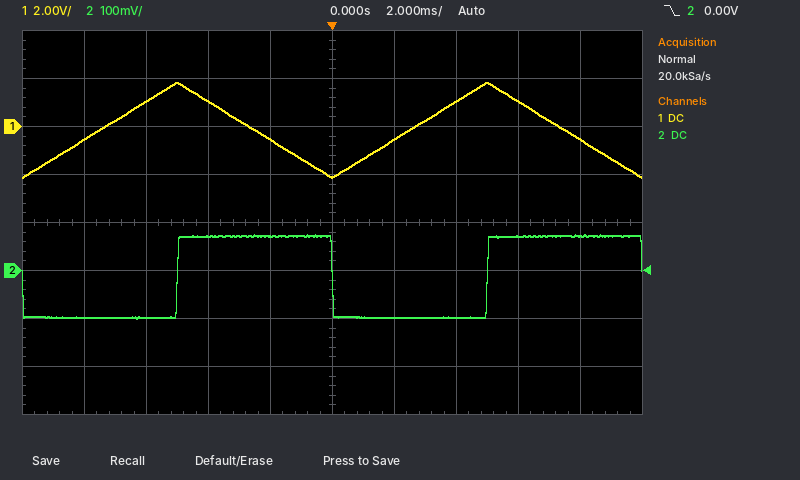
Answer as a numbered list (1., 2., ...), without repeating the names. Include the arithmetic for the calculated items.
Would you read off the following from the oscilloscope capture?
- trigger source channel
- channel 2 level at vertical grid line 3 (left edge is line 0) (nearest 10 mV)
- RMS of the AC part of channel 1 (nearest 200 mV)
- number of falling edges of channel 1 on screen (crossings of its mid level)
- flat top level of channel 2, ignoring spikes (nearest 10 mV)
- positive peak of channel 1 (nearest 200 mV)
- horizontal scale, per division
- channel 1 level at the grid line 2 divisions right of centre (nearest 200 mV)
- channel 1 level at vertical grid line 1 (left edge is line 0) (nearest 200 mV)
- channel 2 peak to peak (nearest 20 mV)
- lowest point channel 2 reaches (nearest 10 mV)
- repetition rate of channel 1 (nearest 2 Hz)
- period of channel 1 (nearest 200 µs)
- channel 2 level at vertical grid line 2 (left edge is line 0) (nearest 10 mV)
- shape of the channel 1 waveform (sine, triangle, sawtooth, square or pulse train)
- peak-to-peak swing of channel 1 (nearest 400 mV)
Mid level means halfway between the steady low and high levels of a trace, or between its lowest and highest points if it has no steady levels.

1. channel 2
2. 70 mV
3. 4.0 V / (2√3) ≈ 1.2 V
4. 2
5. 70 mV
6. 1.8 V
7. 2 ms
8. 1.0 V
9. -600 mV
10. 180 mV
11. -100 mV
12. 1 / 10.0 ms ≈ 100 Hz
13. 10.0 ms
14. -100 mV
15. triangle
16. 4.0 V
